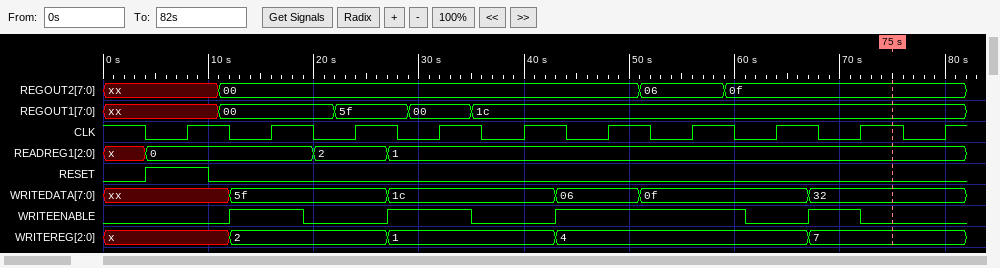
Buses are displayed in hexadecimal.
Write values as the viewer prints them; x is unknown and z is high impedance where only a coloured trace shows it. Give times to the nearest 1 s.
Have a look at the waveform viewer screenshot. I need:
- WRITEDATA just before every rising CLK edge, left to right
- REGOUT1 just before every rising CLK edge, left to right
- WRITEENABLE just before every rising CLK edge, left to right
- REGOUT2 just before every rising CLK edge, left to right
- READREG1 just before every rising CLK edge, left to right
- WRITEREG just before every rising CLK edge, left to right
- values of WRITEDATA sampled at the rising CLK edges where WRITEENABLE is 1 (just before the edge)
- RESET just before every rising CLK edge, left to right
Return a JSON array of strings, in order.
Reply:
["xx, 5f, 5f, 1c, 1c, 06, 0f, 0f, 32, 32", "xx, 00, 5f, 00, 1c, 1c, 1c, 1c, 1c, 1c", "0 1 0 1 0 1 1 0 1 0", "xx, 00, 00, 00, 00, 00, 06, 0f, 0f, 0f", "0, 0, 2, 1, 1, 1, 1, 1, 1, 1", "x, 2, 2, 1, 1, 4, 4, 4, 7, 7", "5f, 1c, 06, 0f, 32", "1 0 0 0 0 0 0 0 0 0"]
